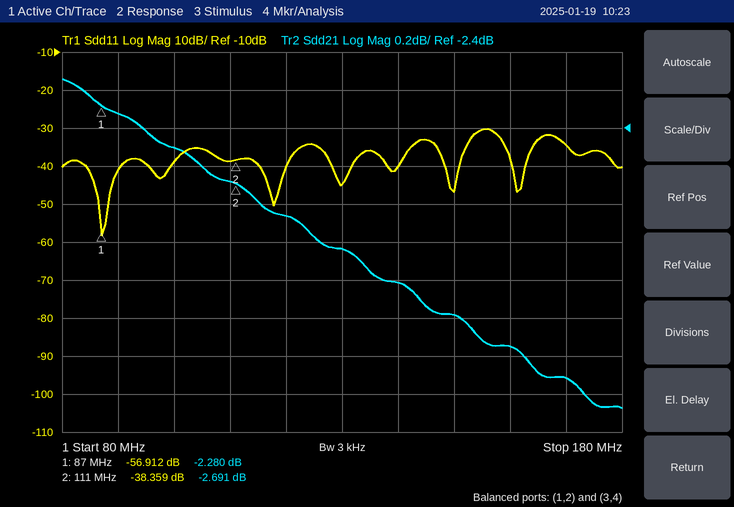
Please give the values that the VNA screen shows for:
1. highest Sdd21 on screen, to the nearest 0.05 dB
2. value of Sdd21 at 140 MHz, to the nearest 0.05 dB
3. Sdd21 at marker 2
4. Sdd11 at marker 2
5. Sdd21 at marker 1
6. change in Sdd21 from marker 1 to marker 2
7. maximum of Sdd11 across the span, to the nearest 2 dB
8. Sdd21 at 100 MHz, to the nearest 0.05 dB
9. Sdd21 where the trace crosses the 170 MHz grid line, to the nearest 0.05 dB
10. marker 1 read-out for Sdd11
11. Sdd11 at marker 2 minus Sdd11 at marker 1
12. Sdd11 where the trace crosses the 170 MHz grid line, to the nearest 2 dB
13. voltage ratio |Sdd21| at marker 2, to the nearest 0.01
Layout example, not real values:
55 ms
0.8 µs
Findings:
-2.15 dB
-3.20 dB
-2.691 dB
-38.359 dB
-2.280 dB
-0.411 dB
-30 dB
-2.50 dB
-3.70 dB
-56.912 dB
18.553 dB
-34 dB
0.73
